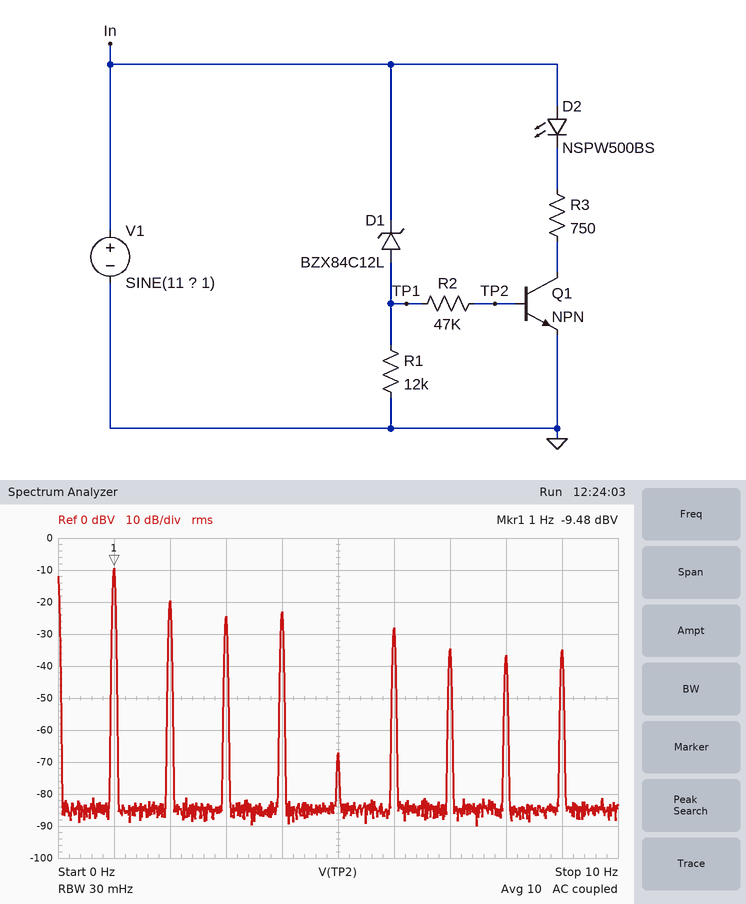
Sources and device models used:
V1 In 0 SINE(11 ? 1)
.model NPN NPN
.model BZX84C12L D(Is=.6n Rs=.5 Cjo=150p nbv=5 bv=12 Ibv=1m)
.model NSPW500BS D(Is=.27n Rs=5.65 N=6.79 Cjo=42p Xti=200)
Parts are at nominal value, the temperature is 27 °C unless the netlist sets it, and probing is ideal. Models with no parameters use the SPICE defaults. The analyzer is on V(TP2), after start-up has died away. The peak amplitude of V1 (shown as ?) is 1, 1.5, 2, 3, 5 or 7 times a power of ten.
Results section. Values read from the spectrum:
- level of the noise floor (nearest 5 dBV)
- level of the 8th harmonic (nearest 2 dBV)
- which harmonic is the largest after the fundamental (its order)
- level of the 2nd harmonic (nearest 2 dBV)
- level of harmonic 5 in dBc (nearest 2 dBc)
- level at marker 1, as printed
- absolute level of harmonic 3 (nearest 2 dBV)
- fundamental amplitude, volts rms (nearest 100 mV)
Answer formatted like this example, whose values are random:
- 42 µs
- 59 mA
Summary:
- -85 dBV
- -36 dBV
- 2
- -20 dBV
- -58 dBc
- -9.48 dBV
- -24 dBV
- 300 mV
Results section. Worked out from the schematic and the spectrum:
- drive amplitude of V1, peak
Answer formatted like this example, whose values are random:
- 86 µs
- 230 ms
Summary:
- 3 V
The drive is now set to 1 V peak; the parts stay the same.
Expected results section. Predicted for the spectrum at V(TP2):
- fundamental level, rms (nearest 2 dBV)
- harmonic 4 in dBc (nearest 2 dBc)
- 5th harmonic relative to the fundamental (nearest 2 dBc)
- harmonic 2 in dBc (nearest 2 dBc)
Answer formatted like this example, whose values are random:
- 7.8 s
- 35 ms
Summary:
- -18 dBV
- -48 dBc
- -28 dBc
- -4 dBc
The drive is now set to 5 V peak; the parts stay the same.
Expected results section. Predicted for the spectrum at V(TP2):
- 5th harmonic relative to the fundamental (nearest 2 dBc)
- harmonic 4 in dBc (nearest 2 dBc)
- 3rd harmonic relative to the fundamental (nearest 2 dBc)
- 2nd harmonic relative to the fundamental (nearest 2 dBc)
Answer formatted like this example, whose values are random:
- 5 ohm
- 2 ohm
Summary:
- -20 dBc
- -16 dBc
- -12 dBc
- -14 dBc
